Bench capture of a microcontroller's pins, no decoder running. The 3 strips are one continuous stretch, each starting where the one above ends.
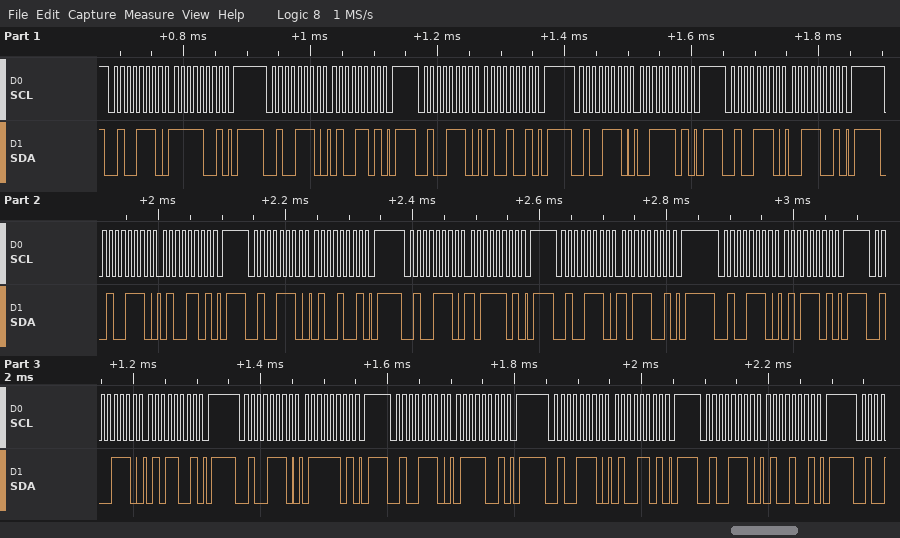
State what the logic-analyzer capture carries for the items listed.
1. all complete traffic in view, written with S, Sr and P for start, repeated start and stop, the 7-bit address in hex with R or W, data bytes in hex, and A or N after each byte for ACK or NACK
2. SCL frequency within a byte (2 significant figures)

S 27W A F9 A P S 27W A 4D A P S 27W A 49 A P S 27W A 3D A P S 27W A 39 A P S 27W A 4D A P S 27W A 49 A P S 27W A BD A P S 27W A B9 A P S 27W A 5D A P S 27W A 59 A P S 27W A 7D A P S 27W A 79 A P S 27W A 4D A P S 27W A 49 A P
100 kHz
